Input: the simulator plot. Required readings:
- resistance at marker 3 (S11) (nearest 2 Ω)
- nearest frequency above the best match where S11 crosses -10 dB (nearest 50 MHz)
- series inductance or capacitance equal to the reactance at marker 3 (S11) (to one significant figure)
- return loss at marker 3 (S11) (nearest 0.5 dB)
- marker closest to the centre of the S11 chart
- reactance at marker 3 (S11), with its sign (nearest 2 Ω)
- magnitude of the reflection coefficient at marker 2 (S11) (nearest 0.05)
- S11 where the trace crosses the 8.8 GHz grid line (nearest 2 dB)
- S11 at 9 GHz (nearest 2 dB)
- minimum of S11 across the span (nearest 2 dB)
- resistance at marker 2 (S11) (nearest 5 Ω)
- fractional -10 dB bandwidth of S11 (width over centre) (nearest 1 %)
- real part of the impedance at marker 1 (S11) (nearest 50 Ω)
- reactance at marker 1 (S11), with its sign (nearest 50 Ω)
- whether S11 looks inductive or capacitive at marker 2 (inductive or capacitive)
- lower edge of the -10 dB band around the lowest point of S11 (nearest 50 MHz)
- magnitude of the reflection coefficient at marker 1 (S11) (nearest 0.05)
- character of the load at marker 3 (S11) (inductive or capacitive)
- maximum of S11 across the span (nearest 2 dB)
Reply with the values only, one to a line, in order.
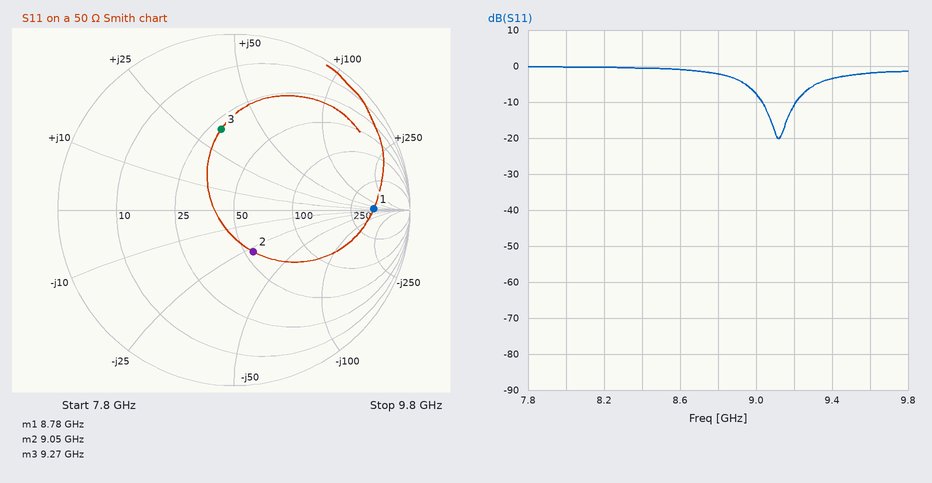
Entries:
28 Ω
9.20 GHz
600 pH
6.5 dB
marker 2
+34 Ω
0.25
-2 dB
-8 dB
-20 dB
55 Ω
2 %
450 Ω
0 Ω
capacitive
9.05 GHz
0.80
inductive
0 dB
